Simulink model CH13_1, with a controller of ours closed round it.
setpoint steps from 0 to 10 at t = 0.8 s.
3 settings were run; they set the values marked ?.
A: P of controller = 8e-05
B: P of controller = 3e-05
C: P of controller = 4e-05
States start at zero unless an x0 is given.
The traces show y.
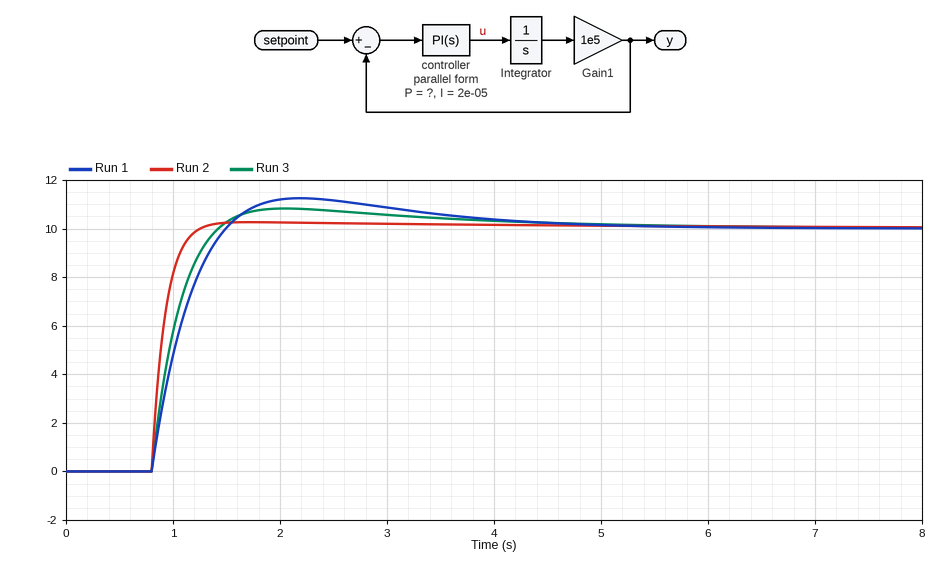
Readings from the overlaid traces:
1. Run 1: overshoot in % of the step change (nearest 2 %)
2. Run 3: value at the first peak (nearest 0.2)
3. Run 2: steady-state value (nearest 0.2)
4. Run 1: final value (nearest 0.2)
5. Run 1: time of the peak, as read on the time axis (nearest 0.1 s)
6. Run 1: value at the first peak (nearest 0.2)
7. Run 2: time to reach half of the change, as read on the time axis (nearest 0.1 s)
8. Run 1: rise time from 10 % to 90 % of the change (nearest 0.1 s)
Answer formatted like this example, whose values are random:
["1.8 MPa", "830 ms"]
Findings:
["12 %", "10.8", "10.0", "10.0", "2.2 s", "11.2", "0.9 s", "0.5 s"]
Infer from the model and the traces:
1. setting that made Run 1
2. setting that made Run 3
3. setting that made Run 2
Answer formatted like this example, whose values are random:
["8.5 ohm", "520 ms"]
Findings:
["B", "C", "A"]
